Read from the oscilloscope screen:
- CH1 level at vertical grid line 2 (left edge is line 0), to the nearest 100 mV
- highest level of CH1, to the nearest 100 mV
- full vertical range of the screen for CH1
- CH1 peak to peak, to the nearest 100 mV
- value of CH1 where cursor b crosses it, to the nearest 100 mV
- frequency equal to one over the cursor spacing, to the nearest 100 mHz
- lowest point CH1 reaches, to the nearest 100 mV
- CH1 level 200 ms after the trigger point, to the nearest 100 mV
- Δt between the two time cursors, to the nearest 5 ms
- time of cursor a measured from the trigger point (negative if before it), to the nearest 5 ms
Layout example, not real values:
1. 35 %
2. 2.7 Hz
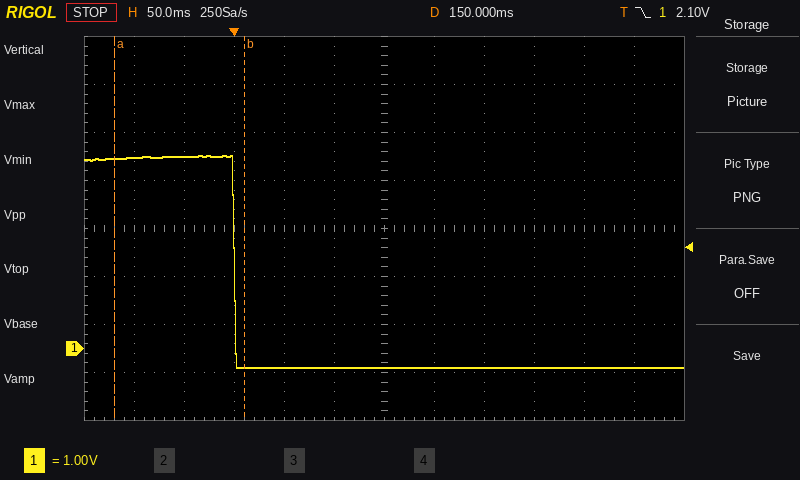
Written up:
1. 4.0 V
2. 4.0 V
3. 8 V
4. 4.4 V
5. -400 mV
6. 7.7 Hz
7. -400 mV
8. -400 mV
9. 130 ms
10. -120 ms
